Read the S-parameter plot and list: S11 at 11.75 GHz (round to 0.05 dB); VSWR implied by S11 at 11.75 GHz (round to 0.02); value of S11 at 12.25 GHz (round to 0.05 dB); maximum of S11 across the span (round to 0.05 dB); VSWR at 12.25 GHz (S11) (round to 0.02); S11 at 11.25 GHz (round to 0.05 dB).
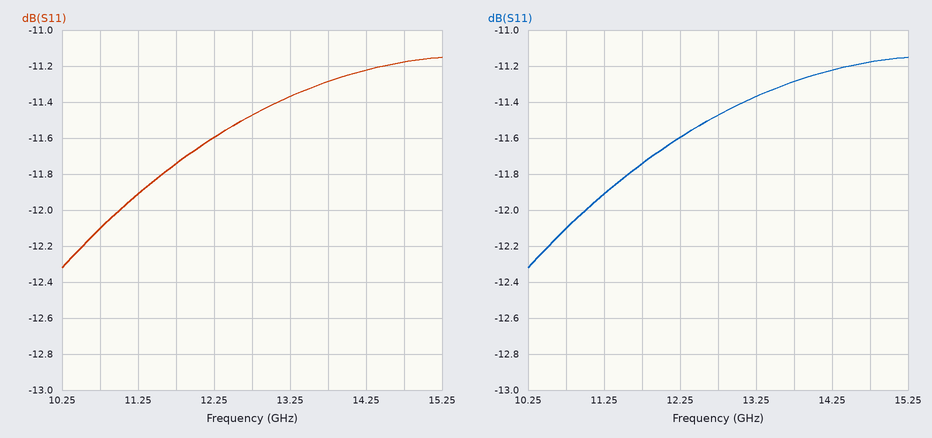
-11.75 dB
1.70
-11.60 dB
-11.15 dB
1.72
-11.90 dB
